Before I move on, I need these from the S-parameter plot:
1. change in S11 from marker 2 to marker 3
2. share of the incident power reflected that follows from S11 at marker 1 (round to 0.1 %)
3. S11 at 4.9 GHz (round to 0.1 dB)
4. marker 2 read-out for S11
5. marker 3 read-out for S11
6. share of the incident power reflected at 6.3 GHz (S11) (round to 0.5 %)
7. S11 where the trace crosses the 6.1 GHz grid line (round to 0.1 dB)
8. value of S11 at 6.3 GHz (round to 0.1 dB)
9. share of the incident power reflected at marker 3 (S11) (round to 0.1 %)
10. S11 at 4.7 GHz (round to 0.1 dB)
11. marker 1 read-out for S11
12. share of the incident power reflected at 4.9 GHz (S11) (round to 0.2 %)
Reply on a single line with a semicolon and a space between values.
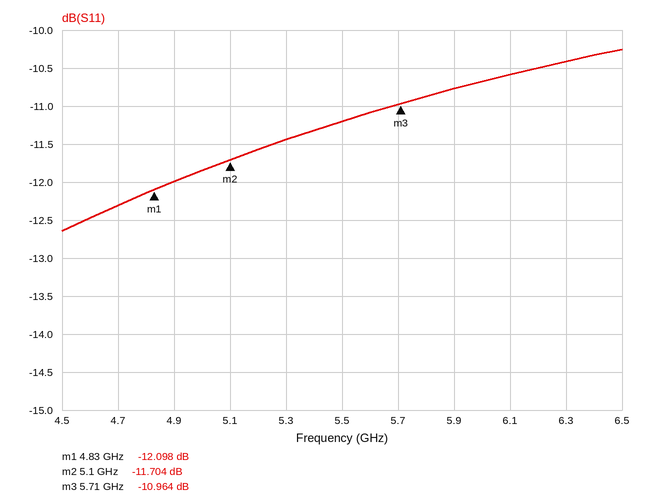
0.740 dB; 6.2 %; -12.0 dB; -11.704 dB; -10.964 dB; 9.0 %; -10.6 dB; -10.4 dB; 8.0 %; -12.3 dB; -12.098 dB; 6.4 %
